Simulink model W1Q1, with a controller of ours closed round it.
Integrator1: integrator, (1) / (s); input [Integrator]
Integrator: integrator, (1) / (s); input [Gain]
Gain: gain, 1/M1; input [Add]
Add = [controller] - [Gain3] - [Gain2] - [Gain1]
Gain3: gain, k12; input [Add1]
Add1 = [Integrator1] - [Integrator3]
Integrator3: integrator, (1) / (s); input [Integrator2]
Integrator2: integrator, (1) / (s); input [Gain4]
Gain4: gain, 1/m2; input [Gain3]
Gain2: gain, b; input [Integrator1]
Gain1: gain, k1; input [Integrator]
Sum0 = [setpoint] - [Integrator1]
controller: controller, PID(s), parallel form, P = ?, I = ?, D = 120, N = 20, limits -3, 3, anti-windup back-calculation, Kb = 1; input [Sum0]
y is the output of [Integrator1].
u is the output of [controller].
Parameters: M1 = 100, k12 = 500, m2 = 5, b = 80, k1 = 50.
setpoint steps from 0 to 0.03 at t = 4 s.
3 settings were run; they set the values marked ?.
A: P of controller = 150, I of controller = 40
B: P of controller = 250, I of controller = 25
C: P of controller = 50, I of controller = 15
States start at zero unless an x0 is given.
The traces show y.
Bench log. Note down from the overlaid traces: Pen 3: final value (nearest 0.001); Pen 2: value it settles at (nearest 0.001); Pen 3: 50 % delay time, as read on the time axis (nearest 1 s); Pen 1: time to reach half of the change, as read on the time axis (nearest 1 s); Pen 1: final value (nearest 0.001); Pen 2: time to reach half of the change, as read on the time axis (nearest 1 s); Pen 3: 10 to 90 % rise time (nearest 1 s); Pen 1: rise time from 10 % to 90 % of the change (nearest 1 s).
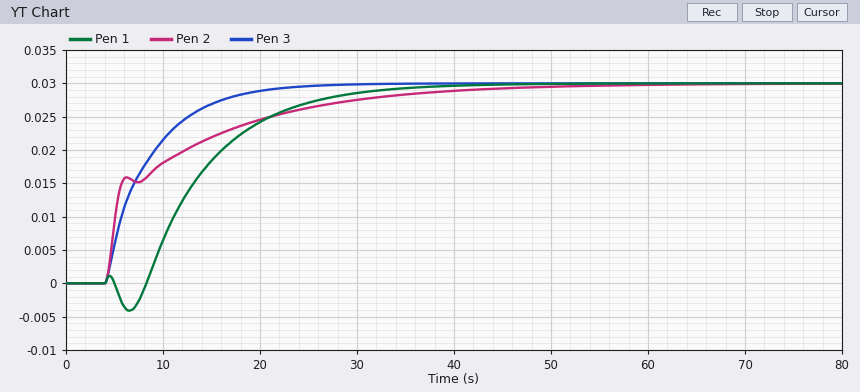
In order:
0.030
0.030
7 s
13 s
0.030
6 s
11 s
16 s
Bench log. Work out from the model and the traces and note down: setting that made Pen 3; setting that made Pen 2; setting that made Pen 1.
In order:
A
B
C
